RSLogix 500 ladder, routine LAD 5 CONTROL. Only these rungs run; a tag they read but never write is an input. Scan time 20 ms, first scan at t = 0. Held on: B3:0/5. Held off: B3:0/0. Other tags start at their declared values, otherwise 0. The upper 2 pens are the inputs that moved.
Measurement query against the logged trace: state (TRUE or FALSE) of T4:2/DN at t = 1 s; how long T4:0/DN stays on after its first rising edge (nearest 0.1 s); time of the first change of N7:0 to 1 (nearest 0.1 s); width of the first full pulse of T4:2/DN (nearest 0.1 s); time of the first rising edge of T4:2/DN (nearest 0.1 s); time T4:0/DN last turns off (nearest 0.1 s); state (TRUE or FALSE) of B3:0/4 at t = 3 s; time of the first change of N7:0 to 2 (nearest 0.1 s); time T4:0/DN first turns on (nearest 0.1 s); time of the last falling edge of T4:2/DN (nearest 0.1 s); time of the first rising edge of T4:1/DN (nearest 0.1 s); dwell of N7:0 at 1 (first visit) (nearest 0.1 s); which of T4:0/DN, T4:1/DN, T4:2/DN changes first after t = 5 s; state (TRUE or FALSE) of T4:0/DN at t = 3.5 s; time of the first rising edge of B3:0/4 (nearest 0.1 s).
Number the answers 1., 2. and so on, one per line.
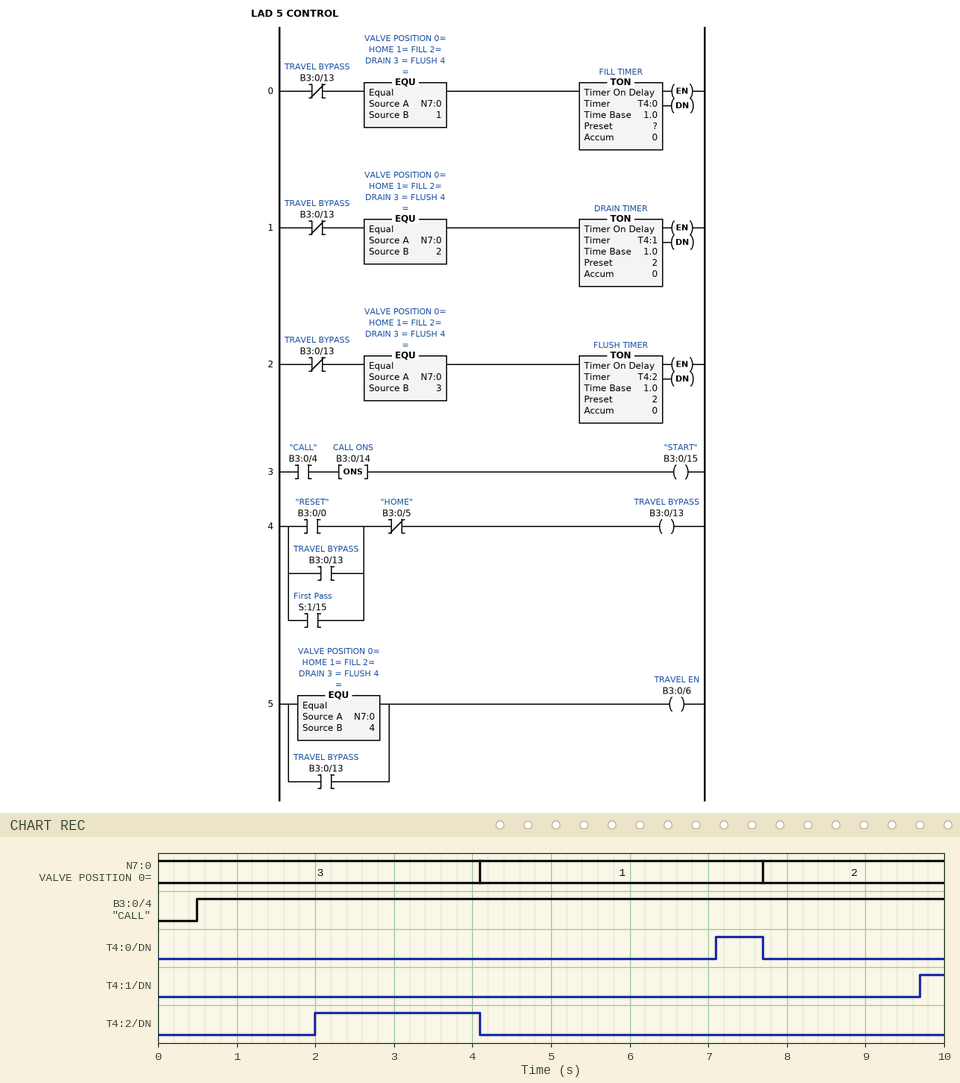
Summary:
1. FALSE
2. 0.6 s
3. 4.1 s
4. 2.1 s
5. 2.0 s
6. 7.7 s
7. TRUE
8. 7.7 s
9. 7.1 s
10. 4.1 s
11. 9.7 s
12. 3.6 s
13. T4:0/DN
14. FALSE
15. 0.5 s
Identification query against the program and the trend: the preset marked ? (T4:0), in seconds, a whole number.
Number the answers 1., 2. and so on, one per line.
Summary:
1. 3 s
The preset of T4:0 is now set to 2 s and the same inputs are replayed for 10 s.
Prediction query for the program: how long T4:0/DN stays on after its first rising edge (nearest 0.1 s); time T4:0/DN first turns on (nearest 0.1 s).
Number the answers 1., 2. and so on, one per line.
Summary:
1. 1.6 s
2. 6.1 s
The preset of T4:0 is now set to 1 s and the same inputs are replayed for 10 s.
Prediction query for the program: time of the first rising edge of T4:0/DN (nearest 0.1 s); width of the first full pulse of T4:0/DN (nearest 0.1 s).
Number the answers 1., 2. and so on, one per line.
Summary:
1. 5.1 s
2. 2.6 s
